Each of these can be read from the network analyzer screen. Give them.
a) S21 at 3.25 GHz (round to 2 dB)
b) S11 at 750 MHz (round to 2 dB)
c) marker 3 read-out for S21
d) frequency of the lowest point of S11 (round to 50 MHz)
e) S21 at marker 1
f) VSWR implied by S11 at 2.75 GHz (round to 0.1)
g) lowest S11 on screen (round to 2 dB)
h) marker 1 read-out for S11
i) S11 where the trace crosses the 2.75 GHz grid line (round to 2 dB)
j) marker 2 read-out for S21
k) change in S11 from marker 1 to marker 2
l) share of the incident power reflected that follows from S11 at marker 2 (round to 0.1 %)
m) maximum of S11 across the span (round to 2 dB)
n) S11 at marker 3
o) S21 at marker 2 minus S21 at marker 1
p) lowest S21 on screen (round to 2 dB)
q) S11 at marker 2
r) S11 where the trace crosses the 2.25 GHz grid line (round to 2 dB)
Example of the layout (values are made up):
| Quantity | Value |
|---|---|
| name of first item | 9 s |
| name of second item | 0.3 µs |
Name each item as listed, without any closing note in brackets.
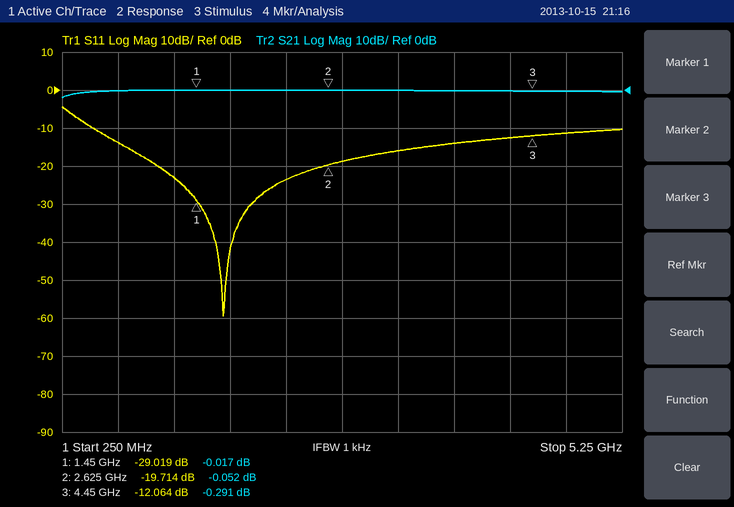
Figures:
| Quantity | Value |
|---|---|
| S21 at 3.25 GHz | 0 dB |
| S11 at 750 MHz | -14 dB |
| marker 3 read-out for S21 | -0.291 dB |
| frequency of the lowest point of S11 | 1.70 GHz |
| S21 at marker 1 | -0.017 dB |
| VSWR implied by S11 at 2.75 GHz | 1.3 |
| lowest S11 on screen | -60 dB |
| marker 1 read-out for S11 | -29.019 dB |
| S11 where the trace crosses the 2.75 GHz grid line | -18 dB |
| marker 2 read-out for S21 | -0.052 dB |
| change in S11 from marker 1 to marker 2 | 9.305 dB |
| share of the incident power reflected that follows from S11 at marker 2 | 1.1 % |
| maximum of S11 across the span | -4 dB |
| S11 at marker 3 | -12.064 dB |
| S21 at marker 2 minus S21 at marker 1 | -0.035 dB |
| lowest S21 on screen | -2 dB |
| S11 at marker 2 | -19.714 dB |
| S11 where the trace crosses the 2.25 GHz grid line | -24 dB |
